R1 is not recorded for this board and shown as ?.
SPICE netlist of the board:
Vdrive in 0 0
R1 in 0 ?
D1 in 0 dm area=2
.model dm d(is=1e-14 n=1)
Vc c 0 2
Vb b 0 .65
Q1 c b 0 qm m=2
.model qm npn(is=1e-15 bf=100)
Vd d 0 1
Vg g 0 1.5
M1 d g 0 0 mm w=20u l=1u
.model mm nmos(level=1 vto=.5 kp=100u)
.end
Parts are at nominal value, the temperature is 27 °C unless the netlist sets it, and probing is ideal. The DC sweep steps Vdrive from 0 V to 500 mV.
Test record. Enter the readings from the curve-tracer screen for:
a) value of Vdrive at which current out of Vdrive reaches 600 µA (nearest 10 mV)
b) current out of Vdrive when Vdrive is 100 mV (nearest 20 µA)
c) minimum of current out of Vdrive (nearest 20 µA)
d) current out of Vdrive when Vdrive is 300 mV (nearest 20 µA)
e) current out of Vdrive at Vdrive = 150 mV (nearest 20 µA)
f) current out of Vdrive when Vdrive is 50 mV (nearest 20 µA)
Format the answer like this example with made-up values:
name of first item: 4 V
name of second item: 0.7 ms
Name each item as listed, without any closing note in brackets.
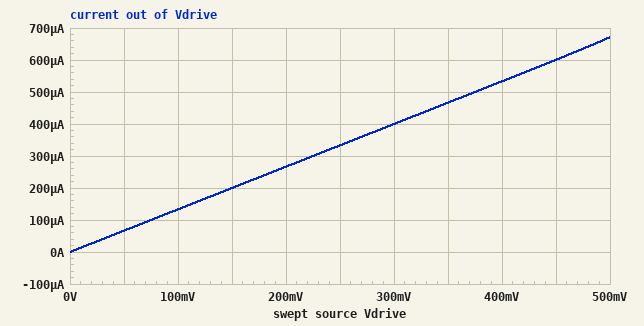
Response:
value of Vdrive at which current out of Vdrive reaches 600 µA: 450 mV
current out of Vdrive when Vdrive is 100 mV: 140 µA
minimum of current out of Vdrive: 0 A
current out of Vdrive when Vdrive is 300 mV: 400 µA
current out of Vdrive at Vdrive = 150 mV: 200 µA
current out of Vdrive when Vdrive is 50 mV: 60 µA
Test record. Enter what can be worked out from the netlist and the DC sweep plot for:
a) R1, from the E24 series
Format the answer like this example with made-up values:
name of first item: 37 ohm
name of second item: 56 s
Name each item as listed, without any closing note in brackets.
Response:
R1, from the E24 series: 750 Ω
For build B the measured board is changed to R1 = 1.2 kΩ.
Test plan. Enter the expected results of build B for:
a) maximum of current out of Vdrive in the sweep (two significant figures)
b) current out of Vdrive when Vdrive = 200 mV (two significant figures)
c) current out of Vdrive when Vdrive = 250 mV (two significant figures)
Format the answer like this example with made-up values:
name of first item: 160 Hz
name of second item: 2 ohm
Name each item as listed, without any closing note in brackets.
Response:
maximum of current out of Vdrive in the sweep: 420 µA
current out of Vdrive when Vdrive = 200 mV: 170 µA
current out of Vdrive when Vdrive = 250 mV: 210 µA
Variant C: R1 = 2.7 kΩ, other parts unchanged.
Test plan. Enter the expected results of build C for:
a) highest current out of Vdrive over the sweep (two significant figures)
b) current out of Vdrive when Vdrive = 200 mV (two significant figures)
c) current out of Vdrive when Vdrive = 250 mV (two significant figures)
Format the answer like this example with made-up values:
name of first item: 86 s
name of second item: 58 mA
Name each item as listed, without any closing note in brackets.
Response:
highest current out of Vdrive over the sweep: 190 µA
current out of Vdrive when Vdrive = 200 mV: 74 µA
current out of Vdrive when Vdrive = 250 mV: 93 µA
